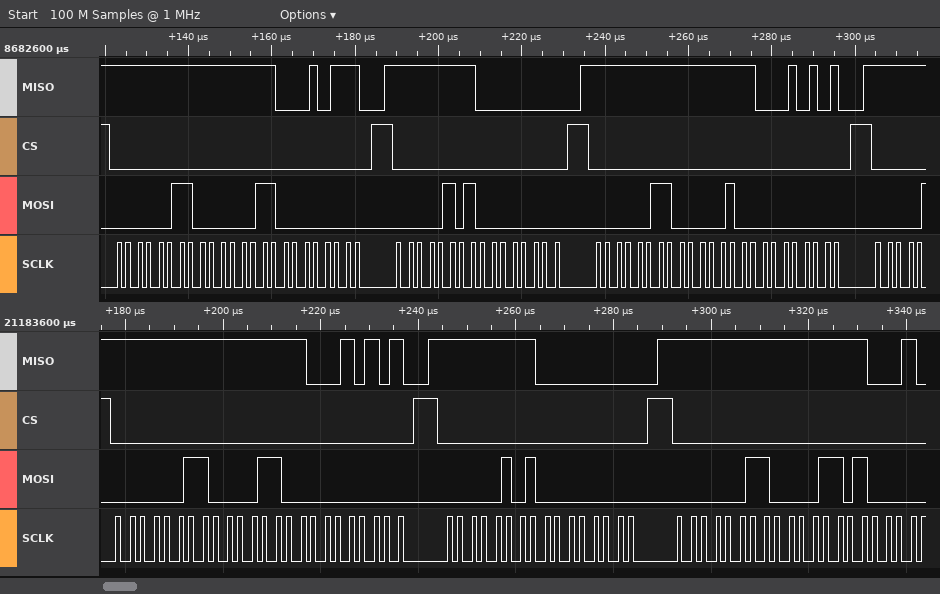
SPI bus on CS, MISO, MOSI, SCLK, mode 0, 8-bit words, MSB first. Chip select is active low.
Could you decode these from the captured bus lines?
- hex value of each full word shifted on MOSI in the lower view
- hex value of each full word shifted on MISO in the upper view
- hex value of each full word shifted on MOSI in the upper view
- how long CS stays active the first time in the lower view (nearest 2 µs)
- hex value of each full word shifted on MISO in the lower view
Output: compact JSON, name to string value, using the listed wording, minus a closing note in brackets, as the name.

{"hex value of each full word shifted on MOSI in the lower view": "03, 0C, 00, 05, 00, 03, 0D", "hex value of each full word shifted on MISO in the upper view": "FF, FF, 17, FF, 00, FF, FF, 15", "hex value of each full word shifted on MOSI in the upper view": "03, 03, 00, 05, 00, 03, 04, 00", "how long CS stays active the first time in the lower view": "62 µs", "hex value of each full word shifted on MISO in the lower view": "FF, FF, 15, FF, 00, FF, FF"}
